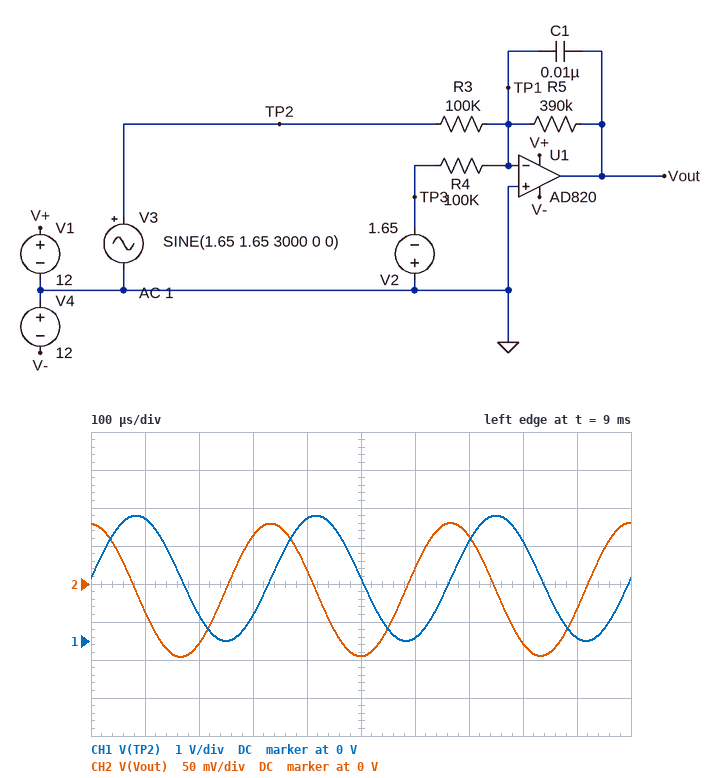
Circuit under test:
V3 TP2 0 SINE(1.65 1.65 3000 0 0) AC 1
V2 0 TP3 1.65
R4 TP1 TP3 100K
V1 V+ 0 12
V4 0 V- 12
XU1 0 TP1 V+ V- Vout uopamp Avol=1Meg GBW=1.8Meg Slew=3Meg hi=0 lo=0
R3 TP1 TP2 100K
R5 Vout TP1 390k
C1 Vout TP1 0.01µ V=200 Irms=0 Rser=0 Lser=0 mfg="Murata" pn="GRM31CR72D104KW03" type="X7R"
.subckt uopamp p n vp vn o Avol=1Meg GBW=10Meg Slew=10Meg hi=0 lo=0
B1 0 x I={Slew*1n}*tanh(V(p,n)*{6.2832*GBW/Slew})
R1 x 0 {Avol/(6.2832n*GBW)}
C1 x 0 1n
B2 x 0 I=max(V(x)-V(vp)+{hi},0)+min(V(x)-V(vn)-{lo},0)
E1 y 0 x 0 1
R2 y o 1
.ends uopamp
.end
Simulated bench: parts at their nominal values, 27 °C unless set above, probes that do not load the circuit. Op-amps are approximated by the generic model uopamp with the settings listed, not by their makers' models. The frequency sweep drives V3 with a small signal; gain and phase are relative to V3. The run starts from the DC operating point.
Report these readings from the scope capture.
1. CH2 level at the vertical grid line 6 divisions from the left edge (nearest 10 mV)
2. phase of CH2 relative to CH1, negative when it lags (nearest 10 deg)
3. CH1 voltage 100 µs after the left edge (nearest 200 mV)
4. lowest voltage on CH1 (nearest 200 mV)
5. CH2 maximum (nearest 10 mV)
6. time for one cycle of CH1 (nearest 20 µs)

20 mV
90 deg
3.2 V
0 V
80 mV
340 µs
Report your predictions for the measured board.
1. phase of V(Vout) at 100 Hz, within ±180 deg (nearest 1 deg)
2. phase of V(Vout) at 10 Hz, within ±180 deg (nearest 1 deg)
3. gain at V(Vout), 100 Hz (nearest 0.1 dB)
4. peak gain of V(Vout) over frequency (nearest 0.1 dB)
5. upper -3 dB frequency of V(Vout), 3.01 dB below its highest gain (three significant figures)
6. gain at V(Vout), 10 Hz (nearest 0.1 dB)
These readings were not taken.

112 deg
166 deg
3.4 dB
11.8 dB
40.8 Hz
11.6 dB
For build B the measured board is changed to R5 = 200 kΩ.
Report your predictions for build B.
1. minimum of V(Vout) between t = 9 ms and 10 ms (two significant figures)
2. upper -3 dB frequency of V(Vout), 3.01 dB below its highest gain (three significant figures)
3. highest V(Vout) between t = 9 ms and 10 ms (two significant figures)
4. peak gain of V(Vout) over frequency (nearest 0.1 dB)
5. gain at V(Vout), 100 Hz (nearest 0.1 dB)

-88 mV
79.6 Hz
87 mV
6.0 dB
1.9 dB
